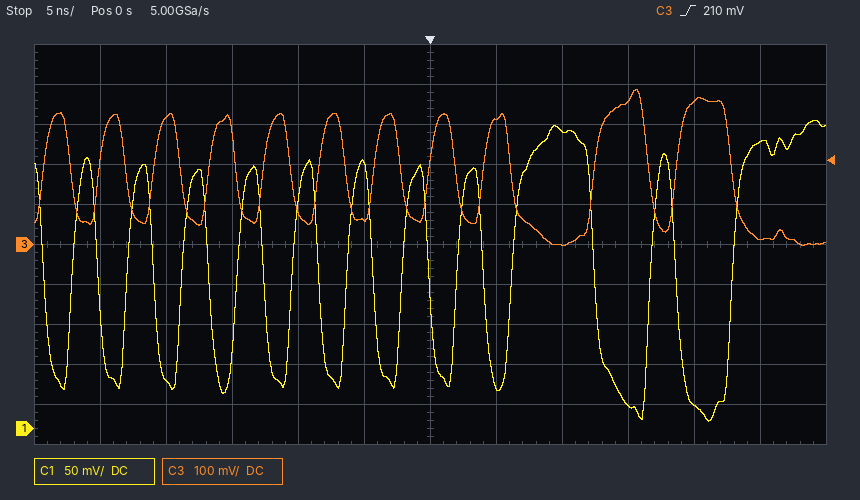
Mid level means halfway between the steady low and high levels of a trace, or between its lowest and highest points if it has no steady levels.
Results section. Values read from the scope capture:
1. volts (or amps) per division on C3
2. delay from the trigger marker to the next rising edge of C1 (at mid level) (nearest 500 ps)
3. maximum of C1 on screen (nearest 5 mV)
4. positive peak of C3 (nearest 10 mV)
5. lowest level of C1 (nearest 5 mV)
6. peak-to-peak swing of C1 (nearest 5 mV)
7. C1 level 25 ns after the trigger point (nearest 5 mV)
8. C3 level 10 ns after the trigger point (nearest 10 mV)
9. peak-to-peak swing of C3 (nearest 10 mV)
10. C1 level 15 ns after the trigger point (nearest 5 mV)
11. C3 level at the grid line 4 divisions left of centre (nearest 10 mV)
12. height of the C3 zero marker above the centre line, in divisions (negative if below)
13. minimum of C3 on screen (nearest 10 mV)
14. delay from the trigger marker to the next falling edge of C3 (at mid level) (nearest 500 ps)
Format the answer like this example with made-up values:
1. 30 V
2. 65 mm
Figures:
1. 100 mV
2. 2.0 ns
3. 385 mV
4. 390 mV
5. 10 mV
6. 375 mV
7. 360 mV
8. 0 mV
9. 390 mV
10. 30 mV
11. 320 mV
12. 0.0 div
13. 0 mV
14. 2.0 ns
